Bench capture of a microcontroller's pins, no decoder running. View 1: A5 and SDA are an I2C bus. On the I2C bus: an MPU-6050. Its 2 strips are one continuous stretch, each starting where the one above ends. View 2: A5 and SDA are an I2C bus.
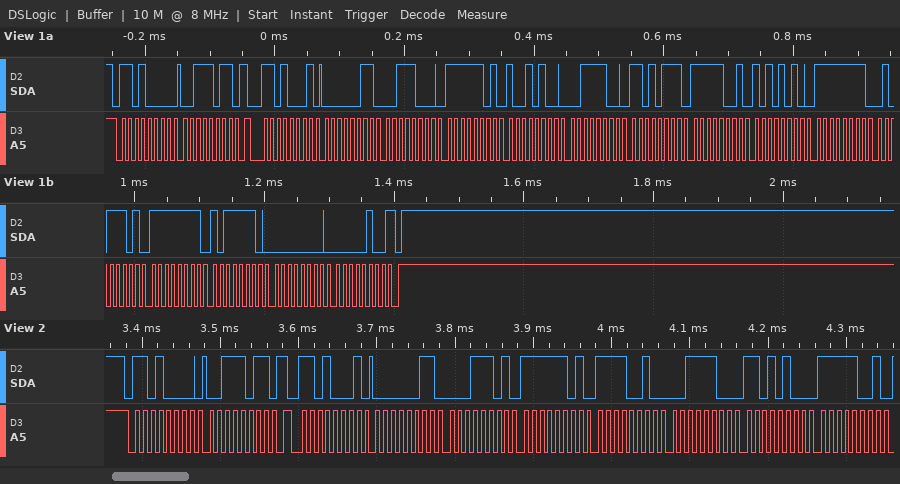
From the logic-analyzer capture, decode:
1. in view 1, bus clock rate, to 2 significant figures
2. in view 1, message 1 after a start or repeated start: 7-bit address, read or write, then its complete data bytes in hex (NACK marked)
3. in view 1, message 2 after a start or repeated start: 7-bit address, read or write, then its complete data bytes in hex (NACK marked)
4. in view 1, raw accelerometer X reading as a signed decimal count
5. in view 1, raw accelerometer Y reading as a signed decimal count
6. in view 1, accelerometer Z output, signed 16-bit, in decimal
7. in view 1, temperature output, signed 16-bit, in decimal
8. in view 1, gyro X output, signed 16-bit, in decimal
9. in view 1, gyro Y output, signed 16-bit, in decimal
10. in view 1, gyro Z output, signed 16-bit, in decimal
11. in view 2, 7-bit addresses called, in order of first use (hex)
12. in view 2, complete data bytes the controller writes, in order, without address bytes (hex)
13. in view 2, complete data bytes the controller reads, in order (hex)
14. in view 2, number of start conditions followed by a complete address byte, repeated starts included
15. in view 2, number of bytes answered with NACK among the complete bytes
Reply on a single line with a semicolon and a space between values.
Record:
100 kHz; 0x68 write: 3B; 0x68 read: 03 38 FD 94 3C D7 F9 AA FF 5D FF BE 00 04 NACK; 824; -620; 15575; -1622; -163; -66; 4; 0x68; 3B; 03 1D FD F2 3C D4 F9; 2; 0
